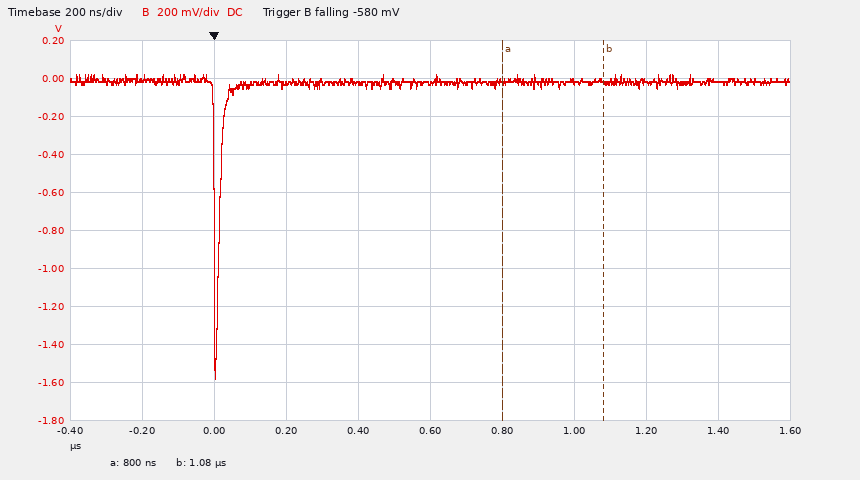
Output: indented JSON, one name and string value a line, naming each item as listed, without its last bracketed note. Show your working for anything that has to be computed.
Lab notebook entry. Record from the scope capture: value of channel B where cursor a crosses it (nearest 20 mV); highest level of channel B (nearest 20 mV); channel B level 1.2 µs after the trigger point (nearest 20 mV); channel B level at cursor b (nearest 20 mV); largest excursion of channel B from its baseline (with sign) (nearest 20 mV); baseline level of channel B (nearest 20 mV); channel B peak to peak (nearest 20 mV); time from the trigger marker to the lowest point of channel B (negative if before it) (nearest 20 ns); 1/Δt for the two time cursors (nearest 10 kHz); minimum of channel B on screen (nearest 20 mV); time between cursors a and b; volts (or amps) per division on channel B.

{
  "value of channel B where cursor a crosses it": "-20 mV",
  "highest level of channel B": "20 mV",
  "channel B level 1.2 µs after the trigger point": "-20 mV",
  "channel B level at cursor b": "-20 mV",
  "largest excursion of channel B from its baseline (with sign)": "-1.58 V − (-20 mV) = -1.56 V",
  "baseline level of channel B": "-20 mV",
  "channel B peak to peak": "20 mV − (-1.58 V) = 1.60 V",
  "time from the trigger marker to the lowest point of channel B (negative if before it)": "0 ns",
  "1/Δt for the two time cursors": "1 / 280 ns ≈ 3.57 MHz",
  "minimum of channel B on screen": "-1.58 V",
  "time between cursors a and b": "1.08 µs − (800 ns) = 280 ns",
  "volts (or amps) per division on channel B": "200 mV"
}
